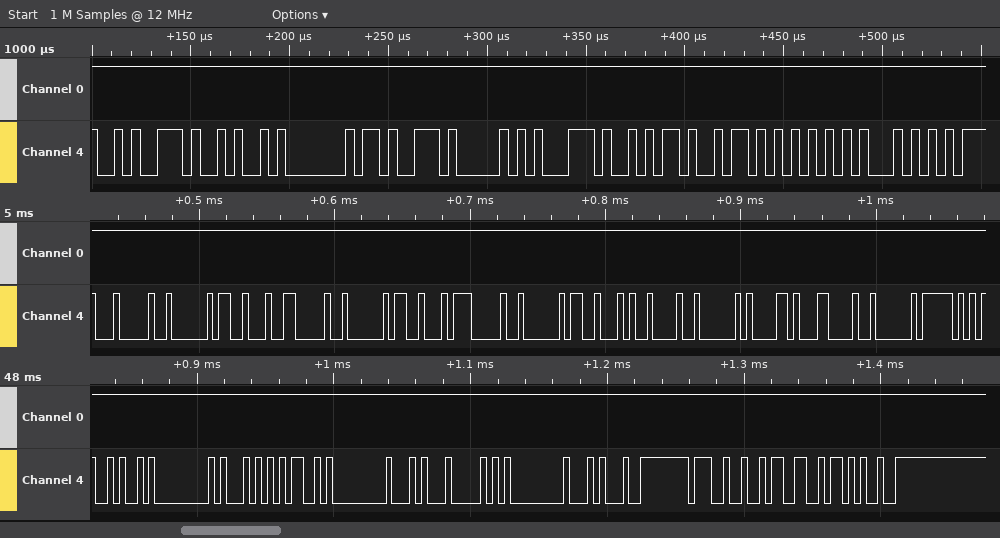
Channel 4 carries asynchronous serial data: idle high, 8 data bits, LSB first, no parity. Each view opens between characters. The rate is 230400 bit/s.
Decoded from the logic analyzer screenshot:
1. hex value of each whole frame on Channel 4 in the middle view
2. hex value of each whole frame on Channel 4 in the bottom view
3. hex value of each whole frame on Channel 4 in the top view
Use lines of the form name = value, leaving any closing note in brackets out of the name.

hex value of each whole frame on Channel 4 in the middle view = 04, 02, 13, 06, 02, 13, 07, 02, 13, 09, 02, 61, 0C, 02, 5F
hex value of each whole frame on Channel 4 in the bottom view = 4A, 00, 51, 4D, 00, 14, 50, 00, 14, FE, 27, 9A, 5A, F2
hex value of each whole frame on Channel 4 in the top view = CA, 29, 01, CB, 41, 71, 6A, 5A, 55, 54
